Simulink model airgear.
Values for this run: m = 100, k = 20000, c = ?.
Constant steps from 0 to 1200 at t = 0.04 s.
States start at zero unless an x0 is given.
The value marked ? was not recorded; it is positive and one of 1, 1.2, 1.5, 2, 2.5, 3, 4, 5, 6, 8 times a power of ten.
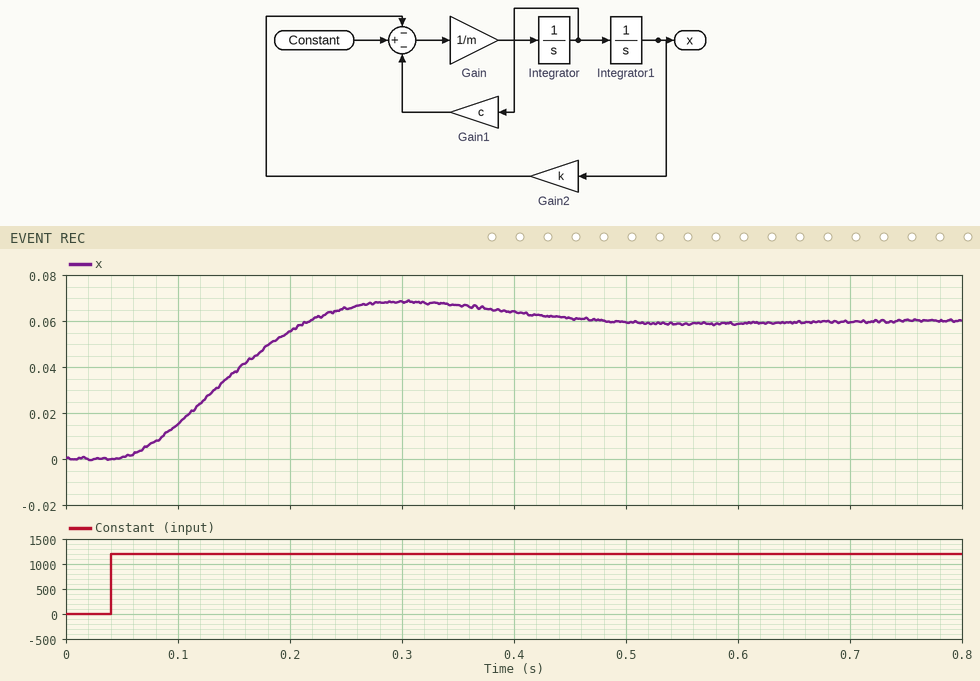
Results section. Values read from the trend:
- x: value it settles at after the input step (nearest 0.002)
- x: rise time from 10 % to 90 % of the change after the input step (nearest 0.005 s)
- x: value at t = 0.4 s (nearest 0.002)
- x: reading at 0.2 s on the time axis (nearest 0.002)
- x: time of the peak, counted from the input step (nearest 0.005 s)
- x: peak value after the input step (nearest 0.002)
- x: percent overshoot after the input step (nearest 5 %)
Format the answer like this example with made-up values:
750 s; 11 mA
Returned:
0.060; 0.120 s; 0.064; 0.056; 0.260 s; 0.068; 15 %
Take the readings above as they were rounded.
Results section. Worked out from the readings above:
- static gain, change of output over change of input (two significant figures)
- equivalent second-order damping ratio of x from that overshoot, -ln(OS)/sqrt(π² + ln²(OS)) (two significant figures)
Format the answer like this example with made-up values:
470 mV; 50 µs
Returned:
0.000050; 0.52
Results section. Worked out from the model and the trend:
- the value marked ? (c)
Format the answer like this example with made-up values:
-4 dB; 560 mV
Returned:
1500
